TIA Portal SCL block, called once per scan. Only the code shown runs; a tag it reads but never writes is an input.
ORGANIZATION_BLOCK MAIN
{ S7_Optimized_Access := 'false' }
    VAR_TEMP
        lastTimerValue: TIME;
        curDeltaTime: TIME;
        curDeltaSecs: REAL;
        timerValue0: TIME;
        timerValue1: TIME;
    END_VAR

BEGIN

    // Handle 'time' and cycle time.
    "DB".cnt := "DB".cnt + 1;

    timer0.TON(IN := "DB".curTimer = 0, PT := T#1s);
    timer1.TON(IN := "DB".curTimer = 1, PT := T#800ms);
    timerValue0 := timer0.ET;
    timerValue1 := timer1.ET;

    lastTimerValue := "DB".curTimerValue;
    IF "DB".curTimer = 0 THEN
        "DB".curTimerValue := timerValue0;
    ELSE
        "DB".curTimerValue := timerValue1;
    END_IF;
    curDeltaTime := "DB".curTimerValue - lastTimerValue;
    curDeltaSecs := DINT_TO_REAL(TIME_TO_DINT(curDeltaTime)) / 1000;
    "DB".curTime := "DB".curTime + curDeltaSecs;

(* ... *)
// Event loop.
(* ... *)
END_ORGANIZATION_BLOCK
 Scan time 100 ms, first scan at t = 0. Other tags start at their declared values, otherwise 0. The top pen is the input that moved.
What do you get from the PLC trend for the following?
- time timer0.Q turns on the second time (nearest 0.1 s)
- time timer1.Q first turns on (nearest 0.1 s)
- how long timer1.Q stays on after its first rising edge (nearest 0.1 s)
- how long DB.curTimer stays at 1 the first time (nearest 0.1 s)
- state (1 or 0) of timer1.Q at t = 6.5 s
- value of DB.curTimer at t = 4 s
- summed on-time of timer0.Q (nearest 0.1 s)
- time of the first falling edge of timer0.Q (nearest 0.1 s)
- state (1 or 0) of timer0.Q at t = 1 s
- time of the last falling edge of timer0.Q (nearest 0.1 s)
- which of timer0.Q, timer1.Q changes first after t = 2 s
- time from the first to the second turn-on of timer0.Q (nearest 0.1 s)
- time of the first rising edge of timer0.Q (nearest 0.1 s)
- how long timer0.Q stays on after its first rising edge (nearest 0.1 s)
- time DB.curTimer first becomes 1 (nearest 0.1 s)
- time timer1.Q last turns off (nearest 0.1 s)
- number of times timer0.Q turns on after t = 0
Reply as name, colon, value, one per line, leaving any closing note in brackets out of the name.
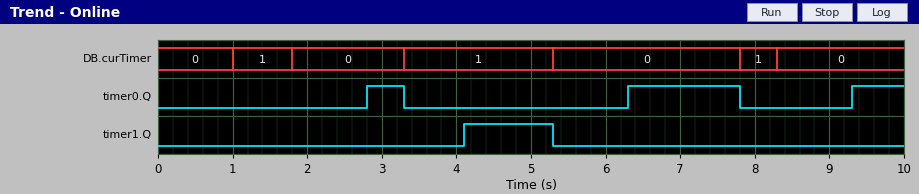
time timer0.Q turns on the second time: 6.3 s
time timer1.Q first turns on: 4.1 s
how long timer1.Q stays on after its first rising edge: 1.2 s
how long DB.curTimer stays at 1 the first time: 0.8 s
state (1 or 0) of timer1.Q at t = 6.5 s: 0
value of DB.curTimer at t = 4 s: 1
summed on-time of timer0.Q: 2.7 s
time of the first falling edge of timer0.Q: 3.3 s
state (1 or 0) of timer0.Q at t = 1 s: 0
time of the last falling edge of timer0.Q: 7.8 s
which of timer0.Q, timer1.Q changes first after t = 2 s: timer0.Q
time from the first to the second turn-on of timer0.Q: 3.5 s
time of the first rising edge of timer0.Q: 2.8 s
how long timer0.Q stays on after its first rising edge: 0.5 s
time DB.curTimer first becomes 1: 1.0 s
time timer1.Q last turns off: 5.3 s
number of times timer0.Q turns on after t = 0: 3
